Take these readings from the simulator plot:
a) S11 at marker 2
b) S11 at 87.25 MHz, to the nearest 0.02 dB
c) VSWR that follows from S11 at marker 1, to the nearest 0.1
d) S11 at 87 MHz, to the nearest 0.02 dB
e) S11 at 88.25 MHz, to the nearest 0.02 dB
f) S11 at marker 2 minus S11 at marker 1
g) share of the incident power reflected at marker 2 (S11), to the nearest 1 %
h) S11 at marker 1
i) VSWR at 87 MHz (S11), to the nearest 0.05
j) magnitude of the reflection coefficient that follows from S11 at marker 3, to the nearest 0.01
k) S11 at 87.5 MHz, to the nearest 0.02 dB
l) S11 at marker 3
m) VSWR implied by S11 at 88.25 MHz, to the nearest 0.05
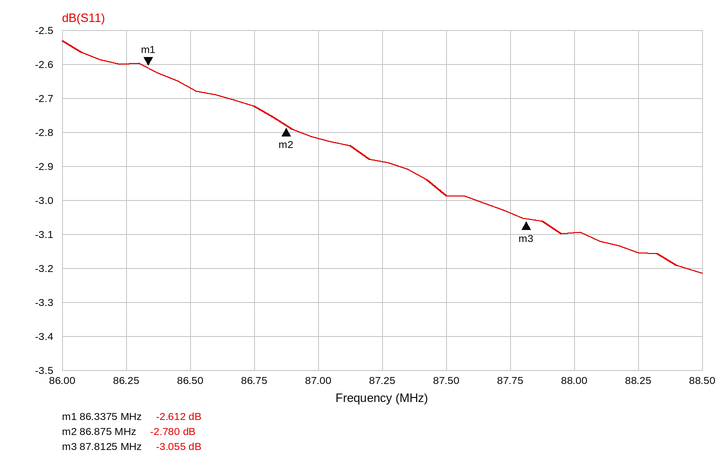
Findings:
-2.780 dB
-2.88 dB
6.7
-2.82 dB
-3.16 dB
-0.168 dB
53 %
-2.612 dB
6.20
0.70
-2.98 dB
-3.055 dB
5.55
